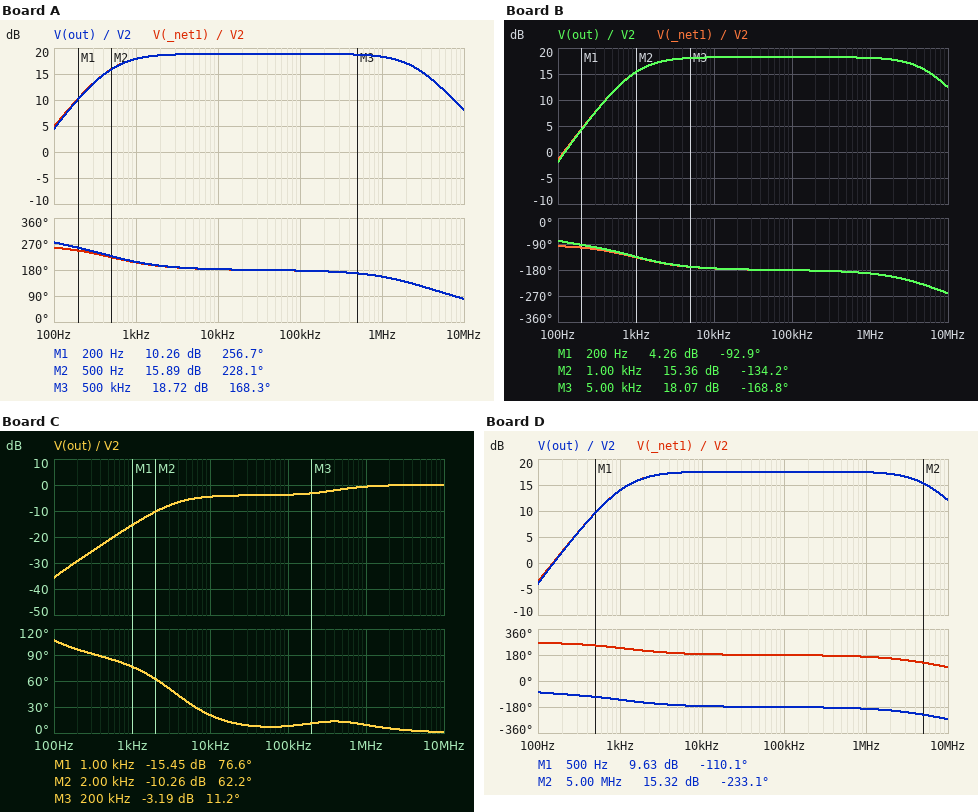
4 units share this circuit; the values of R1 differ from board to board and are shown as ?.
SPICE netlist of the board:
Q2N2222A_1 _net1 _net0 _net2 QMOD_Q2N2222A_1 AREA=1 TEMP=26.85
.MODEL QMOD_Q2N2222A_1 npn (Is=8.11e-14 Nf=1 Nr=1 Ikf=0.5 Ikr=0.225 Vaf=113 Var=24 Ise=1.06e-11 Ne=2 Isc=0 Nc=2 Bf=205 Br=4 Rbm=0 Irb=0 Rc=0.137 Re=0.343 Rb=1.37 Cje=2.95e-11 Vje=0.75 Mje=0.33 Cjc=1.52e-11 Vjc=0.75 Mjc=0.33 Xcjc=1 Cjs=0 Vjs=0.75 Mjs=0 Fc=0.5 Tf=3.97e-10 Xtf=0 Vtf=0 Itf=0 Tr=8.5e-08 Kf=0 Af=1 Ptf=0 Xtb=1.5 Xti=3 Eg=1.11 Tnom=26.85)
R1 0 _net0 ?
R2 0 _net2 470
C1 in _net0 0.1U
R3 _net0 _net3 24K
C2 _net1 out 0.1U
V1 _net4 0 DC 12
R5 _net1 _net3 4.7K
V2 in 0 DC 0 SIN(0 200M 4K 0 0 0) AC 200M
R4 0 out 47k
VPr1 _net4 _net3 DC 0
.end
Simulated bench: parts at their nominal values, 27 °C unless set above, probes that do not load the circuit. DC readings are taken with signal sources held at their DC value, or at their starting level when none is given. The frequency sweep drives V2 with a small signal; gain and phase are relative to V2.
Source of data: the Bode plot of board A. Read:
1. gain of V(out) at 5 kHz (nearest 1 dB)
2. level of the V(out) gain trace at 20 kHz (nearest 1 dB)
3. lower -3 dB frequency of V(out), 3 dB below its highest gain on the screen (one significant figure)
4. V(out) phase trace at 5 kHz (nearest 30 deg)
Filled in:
19 dB
19 dB
500 Hz
180 deg
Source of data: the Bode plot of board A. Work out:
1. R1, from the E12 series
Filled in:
3.9 kΩ
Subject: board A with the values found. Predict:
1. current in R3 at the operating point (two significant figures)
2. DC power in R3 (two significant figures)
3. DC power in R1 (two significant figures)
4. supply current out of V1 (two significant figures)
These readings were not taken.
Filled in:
430 µA
4.5 mW
690 µW
2.6 mA
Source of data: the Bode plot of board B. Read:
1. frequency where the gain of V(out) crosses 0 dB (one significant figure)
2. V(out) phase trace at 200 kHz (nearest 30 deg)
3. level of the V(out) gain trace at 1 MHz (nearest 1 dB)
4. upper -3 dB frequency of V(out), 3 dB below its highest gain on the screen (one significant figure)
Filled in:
100 Hz
-180 deg
18 dB
6 MHz
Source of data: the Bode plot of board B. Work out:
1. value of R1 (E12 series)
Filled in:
1.8 kΩ
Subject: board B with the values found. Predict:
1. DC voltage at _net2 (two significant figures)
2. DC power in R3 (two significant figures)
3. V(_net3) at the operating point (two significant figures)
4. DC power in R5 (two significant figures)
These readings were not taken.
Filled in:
250 mV
5.2 mW
12 V
1.3 mW
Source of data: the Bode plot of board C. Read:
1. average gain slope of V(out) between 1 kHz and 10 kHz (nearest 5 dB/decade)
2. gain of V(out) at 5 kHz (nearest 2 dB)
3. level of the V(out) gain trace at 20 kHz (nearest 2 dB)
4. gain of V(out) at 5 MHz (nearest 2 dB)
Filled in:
10 dB/decade
-6 dB
-4 dB
0 dB
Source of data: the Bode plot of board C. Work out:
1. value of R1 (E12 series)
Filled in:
6.8 kΩ
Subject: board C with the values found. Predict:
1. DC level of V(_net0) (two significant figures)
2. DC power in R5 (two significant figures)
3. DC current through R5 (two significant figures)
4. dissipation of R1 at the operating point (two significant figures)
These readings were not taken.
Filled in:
1.8 V
25 mW
2.3 mA
470 µW
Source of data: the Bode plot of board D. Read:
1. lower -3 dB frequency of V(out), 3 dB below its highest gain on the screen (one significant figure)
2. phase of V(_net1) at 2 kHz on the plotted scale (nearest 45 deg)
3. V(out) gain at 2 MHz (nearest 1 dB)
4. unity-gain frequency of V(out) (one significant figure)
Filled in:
1 kHz
225 deg
17 dB
200 Hz
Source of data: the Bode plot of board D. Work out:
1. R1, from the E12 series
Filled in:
1.5 kΩ
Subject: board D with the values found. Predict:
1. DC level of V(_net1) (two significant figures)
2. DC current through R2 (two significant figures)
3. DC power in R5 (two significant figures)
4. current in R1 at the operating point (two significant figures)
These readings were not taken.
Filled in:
11 V
290 µA
390 µW
470 µA
